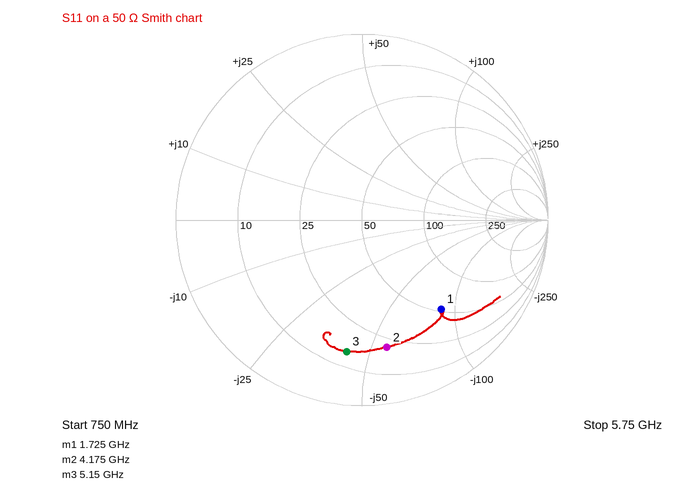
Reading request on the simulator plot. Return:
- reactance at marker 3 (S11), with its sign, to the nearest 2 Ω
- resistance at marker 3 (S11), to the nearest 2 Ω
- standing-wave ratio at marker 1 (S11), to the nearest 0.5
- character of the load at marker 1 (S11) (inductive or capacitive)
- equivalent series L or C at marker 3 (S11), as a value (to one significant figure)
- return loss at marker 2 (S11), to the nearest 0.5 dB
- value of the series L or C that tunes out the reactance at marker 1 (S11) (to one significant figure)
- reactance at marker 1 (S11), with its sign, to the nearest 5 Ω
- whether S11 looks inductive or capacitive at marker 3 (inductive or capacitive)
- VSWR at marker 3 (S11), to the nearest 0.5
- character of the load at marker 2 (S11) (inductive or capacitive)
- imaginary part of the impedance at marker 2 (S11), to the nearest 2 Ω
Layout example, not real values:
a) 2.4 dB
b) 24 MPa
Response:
a) -42 Ω
b) 14 Ω
c) 4.5
d) capacitive
e) 700 fF
f) 3.0 dB
g) 8 nH
h) -85 Ω
i) capacitive
j) 6.0
k) capacitive
l) -56 Ω
